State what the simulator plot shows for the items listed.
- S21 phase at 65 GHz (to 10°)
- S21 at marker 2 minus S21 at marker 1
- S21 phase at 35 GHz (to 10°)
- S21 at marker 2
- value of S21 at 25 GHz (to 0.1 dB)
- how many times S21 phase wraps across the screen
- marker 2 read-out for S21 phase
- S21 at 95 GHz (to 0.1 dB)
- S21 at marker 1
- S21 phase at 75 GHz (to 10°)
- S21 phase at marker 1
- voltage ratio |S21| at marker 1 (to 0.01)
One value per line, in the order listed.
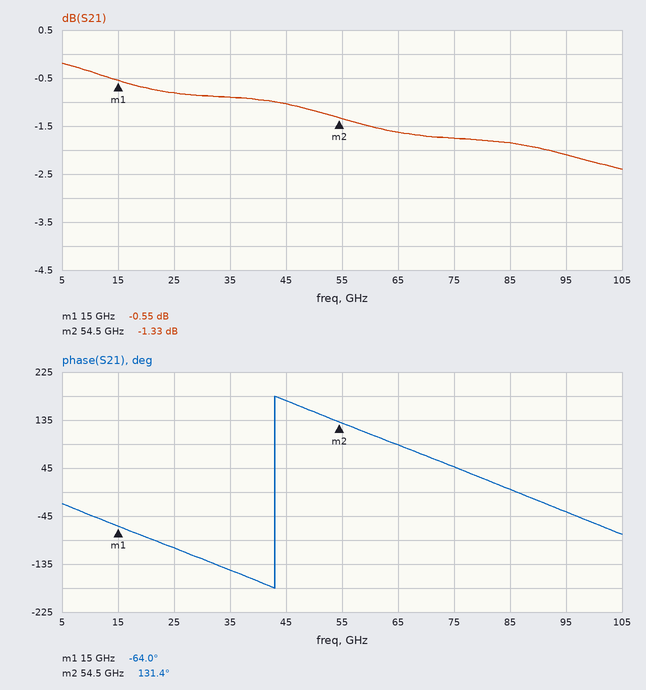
90°
-0.78 dB
-150°
-1.33 dB
-0.8 dB
1
131.4°
-2.1 dB
-0.55 dB
50°
-64.0°
0.94
